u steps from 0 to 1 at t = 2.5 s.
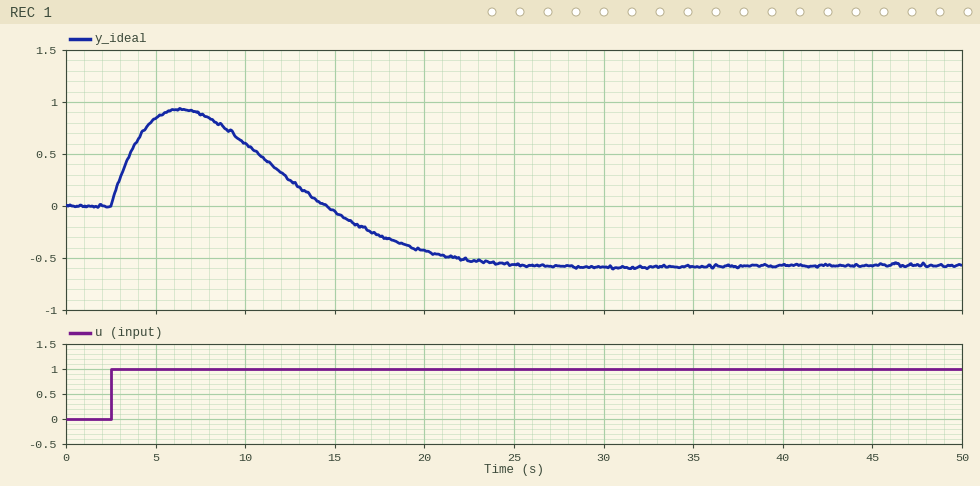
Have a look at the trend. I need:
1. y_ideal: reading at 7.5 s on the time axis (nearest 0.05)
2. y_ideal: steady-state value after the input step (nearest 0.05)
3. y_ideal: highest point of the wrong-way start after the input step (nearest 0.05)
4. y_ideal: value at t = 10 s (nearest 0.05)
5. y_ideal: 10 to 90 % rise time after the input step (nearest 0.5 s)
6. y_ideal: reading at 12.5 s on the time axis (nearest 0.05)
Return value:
0.90
-0.55
0.95
0.60
7.5 s
0.25
